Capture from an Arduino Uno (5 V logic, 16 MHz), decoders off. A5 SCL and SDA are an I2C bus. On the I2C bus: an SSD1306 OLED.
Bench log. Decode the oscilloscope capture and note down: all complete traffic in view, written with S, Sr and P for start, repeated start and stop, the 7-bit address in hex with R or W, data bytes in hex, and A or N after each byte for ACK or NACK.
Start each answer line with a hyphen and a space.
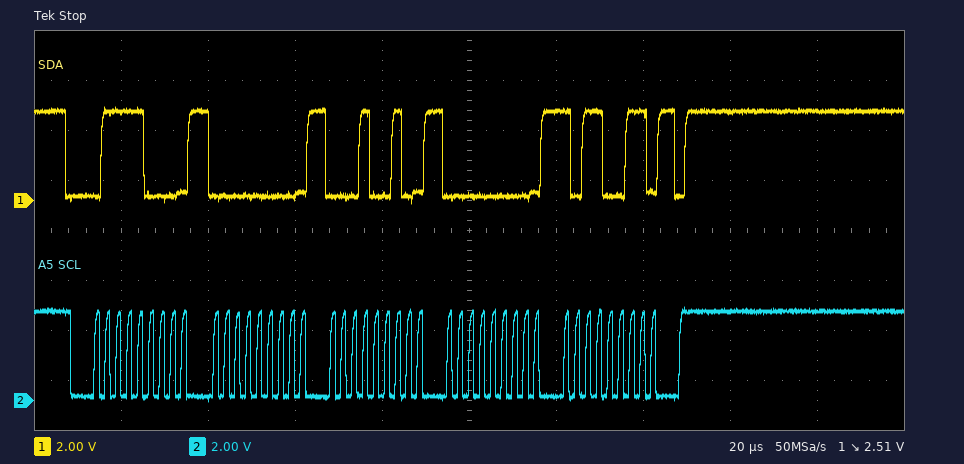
- S 3CW A 00 A 12 A 00 A B3 A P
